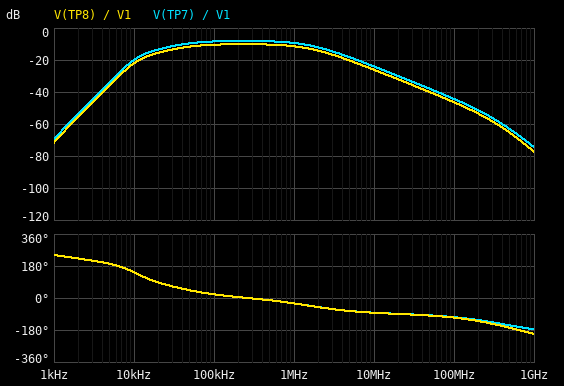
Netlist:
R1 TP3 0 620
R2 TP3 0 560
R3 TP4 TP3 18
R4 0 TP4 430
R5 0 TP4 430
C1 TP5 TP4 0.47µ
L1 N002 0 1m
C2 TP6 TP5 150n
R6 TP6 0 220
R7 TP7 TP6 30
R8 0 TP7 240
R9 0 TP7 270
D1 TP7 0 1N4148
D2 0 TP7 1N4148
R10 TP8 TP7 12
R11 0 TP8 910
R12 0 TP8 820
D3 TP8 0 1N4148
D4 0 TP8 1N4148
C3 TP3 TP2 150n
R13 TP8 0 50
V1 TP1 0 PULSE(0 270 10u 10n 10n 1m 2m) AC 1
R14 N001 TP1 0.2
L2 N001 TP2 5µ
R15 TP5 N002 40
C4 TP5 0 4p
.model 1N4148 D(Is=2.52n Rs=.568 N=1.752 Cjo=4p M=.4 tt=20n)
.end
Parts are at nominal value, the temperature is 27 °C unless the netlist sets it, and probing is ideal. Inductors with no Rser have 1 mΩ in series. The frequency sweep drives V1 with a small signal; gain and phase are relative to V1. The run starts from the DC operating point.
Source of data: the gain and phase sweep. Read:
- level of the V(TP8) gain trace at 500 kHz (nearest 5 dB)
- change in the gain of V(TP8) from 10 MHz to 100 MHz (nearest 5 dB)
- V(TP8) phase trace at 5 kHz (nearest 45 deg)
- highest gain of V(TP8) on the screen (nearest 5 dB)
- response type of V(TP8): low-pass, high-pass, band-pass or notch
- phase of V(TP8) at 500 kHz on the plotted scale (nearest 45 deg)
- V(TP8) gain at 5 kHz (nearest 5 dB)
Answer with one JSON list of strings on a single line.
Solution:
["-10 dB", "-20 dB", "180 deg", "-10 dB", "band-pass", "0 deg", "-35 dB"]
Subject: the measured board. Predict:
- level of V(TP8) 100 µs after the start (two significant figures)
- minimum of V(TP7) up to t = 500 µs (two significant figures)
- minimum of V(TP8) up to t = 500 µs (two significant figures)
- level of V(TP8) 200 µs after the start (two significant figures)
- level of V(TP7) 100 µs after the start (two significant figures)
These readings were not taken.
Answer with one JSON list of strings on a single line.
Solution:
["570 mV", "-1.2 V", "-730 mV", "73 mV", "730 mV"]
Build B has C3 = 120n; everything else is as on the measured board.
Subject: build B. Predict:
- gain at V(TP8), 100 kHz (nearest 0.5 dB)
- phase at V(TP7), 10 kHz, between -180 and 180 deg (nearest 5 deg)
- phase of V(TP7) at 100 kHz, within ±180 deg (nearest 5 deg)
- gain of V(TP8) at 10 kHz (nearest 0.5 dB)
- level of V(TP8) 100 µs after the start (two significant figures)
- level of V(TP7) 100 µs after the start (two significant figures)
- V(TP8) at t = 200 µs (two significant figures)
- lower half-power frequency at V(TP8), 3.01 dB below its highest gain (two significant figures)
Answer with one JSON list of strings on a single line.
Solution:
["-10.5 dB", "150 deg", "25 deg", "-23.5 dB", "530 mV", "680 mV", "56 mV", "37 kHz"]
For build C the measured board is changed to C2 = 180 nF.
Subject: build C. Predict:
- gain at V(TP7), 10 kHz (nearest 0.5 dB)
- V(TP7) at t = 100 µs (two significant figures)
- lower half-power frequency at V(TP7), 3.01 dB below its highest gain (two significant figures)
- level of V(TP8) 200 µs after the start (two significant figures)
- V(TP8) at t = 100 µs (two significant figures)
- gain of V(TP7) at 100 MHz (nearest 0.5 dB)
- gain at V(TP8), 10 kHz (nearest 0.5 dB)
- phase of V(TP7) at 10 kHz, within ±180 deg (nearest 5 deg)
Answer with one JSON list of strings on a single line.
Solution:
["-19.5 dB", "760 mV", "30 kHz", "70 mV", "590 mV", "-44.5 dB", "-21.5 dB", "140 deg"]
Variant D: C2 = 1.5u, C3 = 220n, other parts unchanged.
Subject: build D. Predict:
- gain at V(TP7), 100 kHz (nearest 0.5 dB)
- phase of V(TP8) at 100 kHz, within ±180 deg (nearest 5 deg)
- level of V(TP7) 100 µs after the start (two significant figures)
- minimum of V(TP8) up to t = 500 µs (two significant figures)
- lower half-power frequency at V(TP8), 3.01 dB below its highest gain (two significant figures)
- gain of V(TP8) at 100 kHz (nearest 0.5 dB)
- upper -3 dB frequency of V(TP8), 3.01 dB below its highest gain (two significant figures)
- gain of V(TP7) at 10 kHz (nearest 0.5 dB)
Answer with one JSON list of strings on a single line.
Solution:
["-8.0 dB", "10 deg", "-800 mV", "-720 mV", "18 kHz", "-10.0 dB", "1.6 MHz", "-16.0 dB"]
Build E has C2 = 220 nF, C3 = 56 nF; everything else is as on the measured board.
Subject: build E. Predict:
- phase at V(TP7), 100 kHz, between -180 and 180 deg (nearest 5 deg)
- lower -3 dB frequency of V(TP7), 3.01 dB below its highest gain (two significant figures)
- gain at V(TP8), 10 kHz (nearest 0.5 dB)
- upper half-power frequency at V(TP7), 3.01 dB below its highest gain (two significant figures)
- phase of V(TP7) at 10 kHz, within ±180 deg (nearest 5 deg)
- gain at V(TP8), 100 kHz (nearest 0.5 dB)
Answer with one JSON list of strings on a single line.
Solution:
["35 deg", "61 kHz", "-28.5 dB", "1.7 MHz", "150 deg", "-11.5 dB"]
